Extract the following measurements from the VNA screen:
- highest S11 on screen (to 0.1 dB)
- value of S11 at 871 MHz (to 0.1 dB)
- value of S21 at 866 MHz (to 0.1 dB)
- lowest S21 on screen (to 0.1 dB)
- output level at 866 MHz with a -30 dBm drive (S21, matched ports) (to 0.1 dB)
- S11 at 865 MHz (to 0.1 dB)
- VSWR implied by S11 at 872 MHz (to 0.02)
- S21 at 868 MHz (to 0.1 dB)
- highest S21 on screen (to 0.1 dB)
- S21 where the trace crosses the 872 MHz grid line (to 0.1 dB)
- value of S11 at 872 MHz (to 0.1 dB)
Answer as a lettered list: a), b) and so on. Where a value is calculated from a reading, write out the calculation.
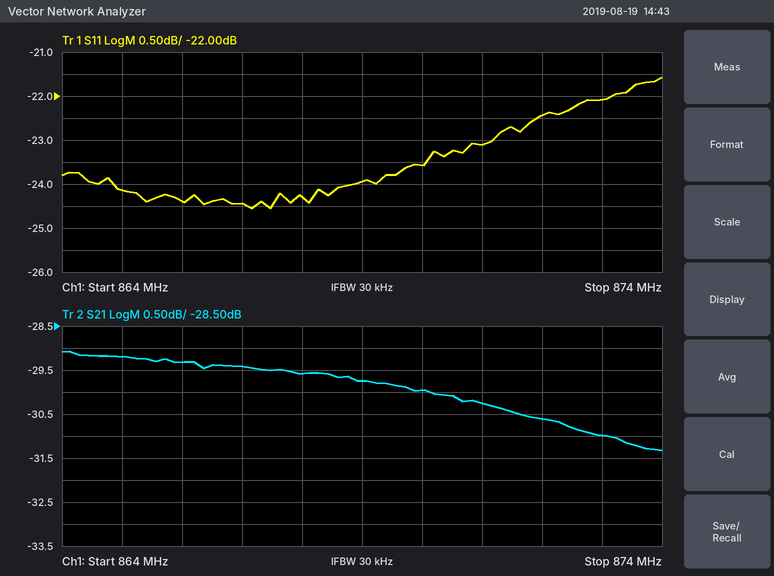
a) -21.6 dB
b) -23.1 dB
c) -29.3 dB
d) -31.3 dB
e) -30 dBm + (-29.3 dB) = -59.3 dBm
f) -24.1 dB
g) |Γ| = 10^(-22.4/20) = 0.0759; VSWR = (1 + 0.0759)/(1 − 0.0759) ≈ 1.16
h) -29.6 dB
i) -29.1 dB
j) -30.6 dB
k) -22.4 dB
